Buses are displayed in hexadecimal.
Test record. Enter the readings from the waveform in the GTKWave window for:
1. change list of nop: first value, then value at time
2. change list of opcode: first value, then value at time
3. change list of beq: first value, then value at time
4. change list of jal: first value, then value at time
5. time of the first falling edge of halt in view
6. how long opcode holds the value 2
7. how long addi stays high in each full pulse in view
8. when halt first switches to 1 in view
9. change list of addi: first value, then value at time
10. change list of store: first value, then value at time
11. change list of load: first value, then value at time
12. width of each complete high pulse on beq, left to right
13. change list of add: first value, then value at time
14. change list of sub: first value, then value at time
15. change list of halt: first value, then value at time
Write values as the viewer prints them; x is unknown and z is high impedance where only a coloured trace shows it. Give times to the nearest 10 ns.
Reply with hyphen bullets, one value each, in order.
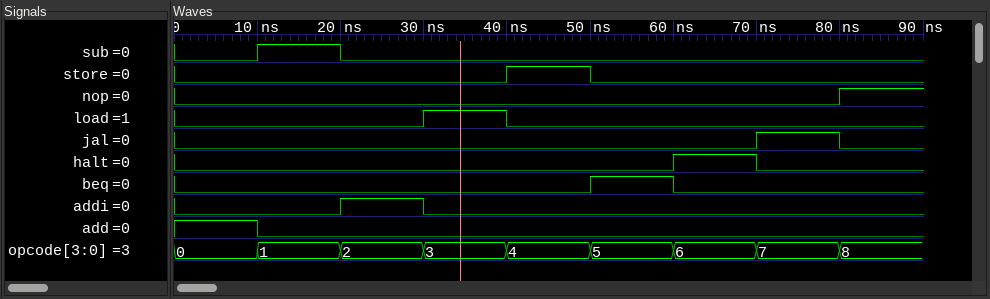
- 0, 1 at 80 ns
- 0, 1 at 10 ns, 2 at 20 ns, 3 at 30 ns, 4 at 40 ns, 5 at 50 ns, 6 at 60 ns, 7 at 70 ns, 8 at 80 ns
- 0, 1 at 50 ns, 0 at 60 ns
- 0, 1 at 70 ns, 0 at 80 ns
- 70 ns
- 10 ns
- 10 ns
- 60 ns
- 0, 1 at 20 ns, 0 at 30 ns
- 0, 1 at 40 ns, 0 at 50 ns
- 0, 1 at 30 ns, 0 at 40 ns
- 10 ns
- 1, 0 at 10 ns
- 0, 1 at 10 ns, 0 at 20 ns
- 0, 1 at 60 ns, 0 at 70 ns
